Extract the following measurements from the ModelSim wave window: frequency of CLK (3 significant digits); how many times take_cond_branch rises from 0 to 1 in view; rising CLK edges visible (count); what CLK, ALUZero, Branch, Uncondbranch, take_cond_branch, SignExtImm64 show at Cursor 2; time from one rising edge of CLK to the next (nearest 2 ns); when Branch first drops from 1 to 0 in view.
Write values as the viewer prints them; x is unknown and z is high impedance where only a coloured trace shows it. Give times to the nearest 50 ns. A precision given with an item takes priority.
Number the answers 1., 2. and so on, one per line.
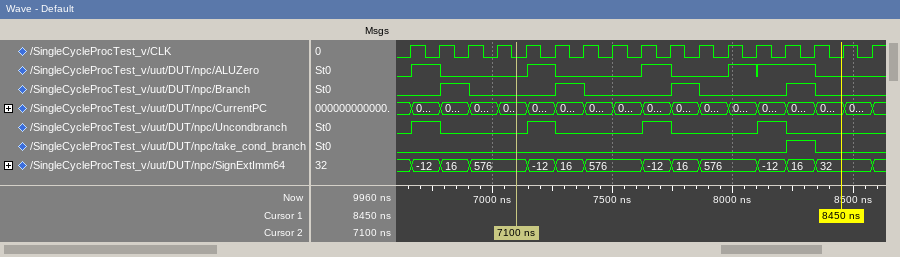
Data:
1. 8.33 MHz
2. 1
3. 17
4. CLK=0, ALUZero=0, Branch=0, Uncondbranch=0, take_cond_branch=0, SignExtImm64=576
5. 120 ns
6. 6900 ns
